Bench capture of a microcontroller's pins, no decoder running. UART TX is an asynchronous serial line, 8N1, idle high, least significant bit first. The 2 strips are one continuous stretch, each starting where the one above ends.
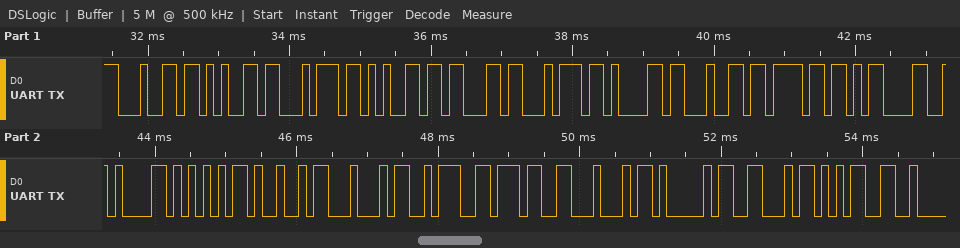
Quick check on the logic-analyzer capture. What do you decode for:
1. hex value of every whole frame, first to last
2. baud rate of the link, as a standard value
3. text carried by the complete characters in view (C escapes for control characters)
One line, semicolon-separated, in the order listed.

64 65 74 65 63 74 61 64 6F 0D 0A 55 49 44 3A 37 44 41 46 35; 9600 baud; "detectado\r\nUID:7DAF5"
